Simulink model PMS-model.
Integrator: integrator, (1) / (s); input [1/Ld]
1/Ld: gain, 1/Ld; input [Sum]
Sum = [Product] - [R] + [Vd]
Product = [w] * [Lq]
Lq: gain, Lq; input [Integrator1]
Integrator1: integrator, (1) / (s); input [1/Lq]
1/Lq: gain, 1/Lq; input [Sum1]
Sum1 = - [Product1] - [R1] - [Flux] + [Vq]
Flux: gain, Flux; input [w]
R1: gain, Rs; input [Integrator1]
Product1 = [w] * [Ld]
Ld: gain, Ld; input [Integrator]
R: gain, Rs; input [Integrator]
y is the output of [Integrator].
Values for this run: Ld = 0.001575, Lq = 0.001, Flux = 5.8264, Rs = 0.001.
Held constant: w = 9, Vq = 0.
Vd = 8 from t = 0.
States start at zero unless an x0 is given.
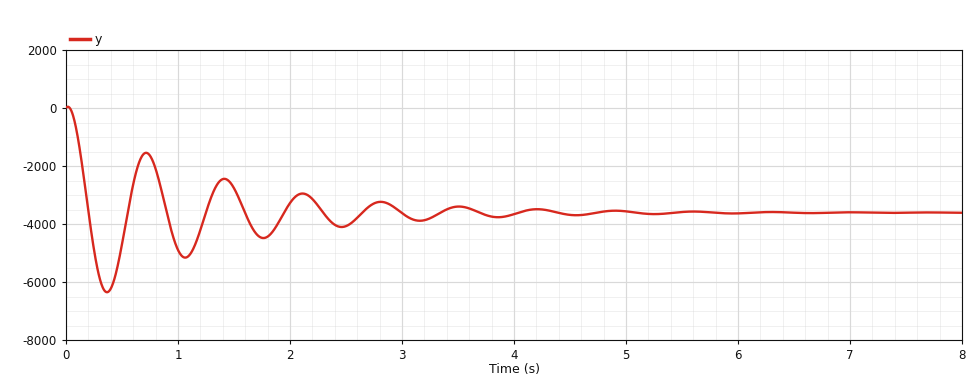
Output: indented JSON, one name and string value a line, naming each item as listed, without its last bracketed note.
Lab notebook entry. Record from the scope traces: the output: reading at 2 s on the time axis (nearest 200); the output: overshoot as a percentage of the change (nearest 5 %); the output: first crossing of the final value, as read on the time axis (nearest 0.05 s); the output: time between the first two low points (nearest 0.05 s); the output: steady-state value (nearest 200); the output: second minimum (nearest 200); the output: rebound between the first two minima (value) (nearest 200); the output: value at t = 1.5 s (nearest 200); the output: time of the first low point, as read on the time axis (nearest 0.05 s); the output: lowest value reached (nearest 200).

{
  "the output: reading at 2 s on the time axis": "-3200",
  "the output: overshoot as a percentage of the change": "75 %",
  "the output: first crossing of the final value, as read on the time axis": "0.20 s",
  "the output: time between the first two low points": "0.70 s",
  "the output: steady-state value": "-3600",
  "the output: second minimum": "-5200",
  "the output: rebound between the first two minima (value)": "-1600",
  "the output: value at t = 1.5 s": "-2800",
  "the output: time of the first low point, as read on the time axis": "0.35 s",
  "the output: lowest value reached": "-6400"
}
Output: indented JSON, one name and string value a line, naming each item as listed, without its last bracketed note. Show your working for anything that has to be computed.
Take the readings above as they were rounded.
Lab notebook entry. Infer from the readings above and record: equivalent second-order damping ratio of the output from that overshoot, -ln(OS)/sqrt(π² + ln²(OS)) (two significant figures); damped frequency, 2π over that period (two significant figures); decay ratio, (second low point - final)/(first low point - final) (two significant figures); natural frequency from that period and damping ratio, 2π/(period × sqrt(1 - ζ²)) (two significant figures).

{
  "equivalent second-order damping ratio of the output from that overshoot, -ln(OS)/sqrt(π² + ln²(OS))": "ln(0.75) = -0.288; 0.288 / sqrt(9.870 + 0.083) = 0.091",
  "damped frequency, 2π over that period": "2π / 0.7 = 9.0 rad/s",
  "decay ratio, (second low point - final)/(first low point - final)": "(-5200 - (-3600)) / (-6400 - (-3600)) = 0.57",
  "natural frequency from that period and damping ratio, 2π/(period × sqrt(1 - ζ²))": "2π / (0.7 × sqrt(1 - 0.091²)) = 9.0 rad/s"
}
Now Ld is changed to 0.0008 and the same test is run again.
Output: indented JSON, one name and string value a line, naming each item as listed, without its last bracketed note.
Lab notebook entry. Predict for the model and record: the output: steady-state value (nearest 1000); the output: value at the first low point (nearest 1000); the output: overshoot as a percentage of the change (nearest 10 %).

{
  "the output: steady-state value": "-7000",
  "the output: value at the first low point": "-12000",
  "the output: overshoot as a percentage of the change": "70 %"
}
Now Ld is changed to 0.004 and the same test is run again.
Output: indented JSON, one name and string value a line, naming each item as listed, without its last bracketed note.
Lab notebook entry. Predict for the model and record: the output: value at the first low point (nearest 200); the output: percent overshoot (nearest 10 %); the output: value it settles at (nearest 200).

{
  "the output: value at the first low point": "-2600",
  "the output: percent overshoot": "80 %",
  "the output: value it settles at": "-1400"
}
